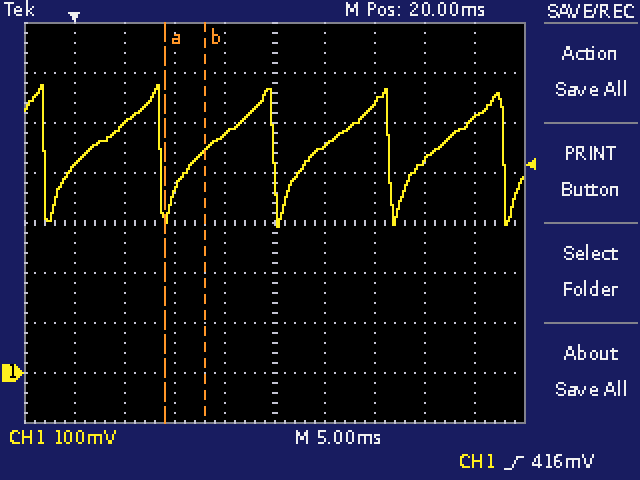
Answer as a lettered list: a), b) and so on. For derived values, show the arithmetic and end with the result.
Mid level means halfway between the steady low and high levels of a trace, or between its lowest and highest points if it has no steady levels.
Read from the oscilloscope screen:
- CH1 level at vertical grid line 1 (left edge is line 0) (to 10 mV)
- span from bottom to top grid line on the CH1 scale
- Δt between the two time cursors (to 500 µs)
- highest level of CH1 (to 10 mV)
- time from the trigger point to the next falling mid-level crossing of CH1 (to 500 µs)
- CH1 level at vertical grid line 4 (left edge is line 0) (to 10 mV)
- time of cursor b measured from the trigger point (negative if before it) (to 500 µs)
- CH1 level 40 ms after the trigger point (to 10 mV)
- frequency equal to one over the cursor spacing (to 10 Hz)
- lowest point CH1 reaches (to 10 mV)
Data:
a) 410 mV
b) 800 mV
c) 4.0 ms
d) 580 mV
e) 8.5 ms
f) 480 mV
g) +13.0 ms
h) 510 mV
i) 1 / 4.0 ms ≈ 250 Hz
j) 290 mV
